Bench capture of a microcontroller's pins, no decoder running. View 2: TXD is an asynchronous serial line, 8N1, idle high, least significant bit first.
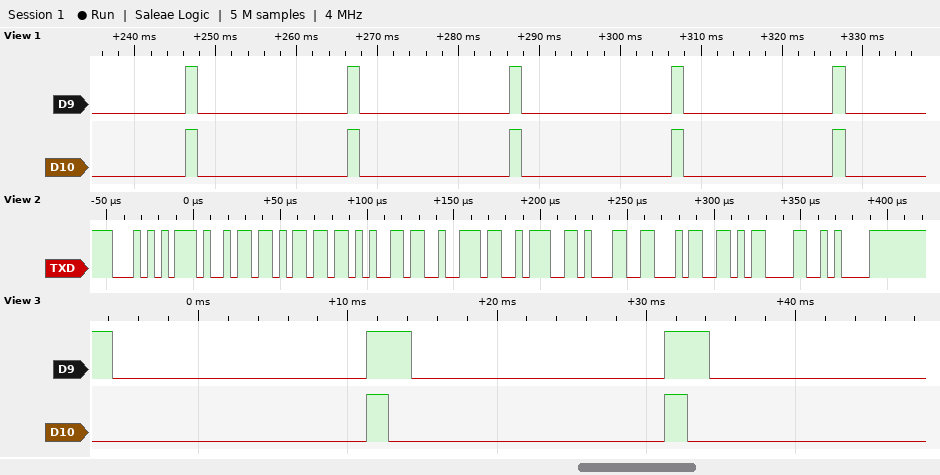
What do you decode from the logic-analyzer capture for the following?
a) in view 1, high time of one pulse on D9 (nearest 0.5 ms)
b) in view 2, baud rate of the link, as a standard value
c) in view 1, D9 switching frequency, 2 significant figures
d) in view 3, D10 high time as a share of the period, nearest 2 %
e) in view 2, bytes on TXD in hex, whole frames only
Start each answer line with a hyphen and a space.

- 1.5 ms
- 250000 baud
- 50 Hz
- 8 %
- 54 69 6D 65 72 3A 31 34 0D 0A
